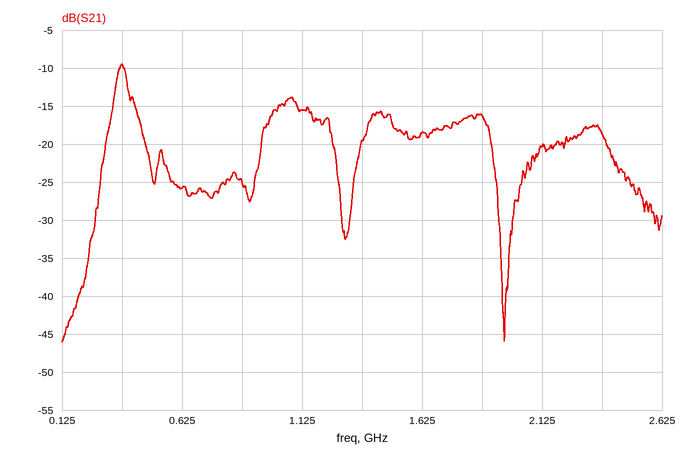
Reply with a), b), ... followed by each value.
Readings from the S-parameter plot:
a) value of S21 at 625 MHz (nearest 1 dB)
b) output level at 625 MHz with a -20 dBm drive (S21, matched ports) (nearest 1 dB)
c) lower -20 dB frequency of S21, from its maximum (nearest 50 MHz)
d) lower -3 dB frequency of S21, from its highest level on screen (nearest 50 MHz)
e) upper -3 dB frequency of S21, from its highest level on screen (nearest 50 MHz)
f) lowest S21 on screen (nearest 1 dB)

a) -26 dB
b) -46 dBm
c) 250 MHz
d) 350 MHz
e) 400 MHz
f) -46 dB
